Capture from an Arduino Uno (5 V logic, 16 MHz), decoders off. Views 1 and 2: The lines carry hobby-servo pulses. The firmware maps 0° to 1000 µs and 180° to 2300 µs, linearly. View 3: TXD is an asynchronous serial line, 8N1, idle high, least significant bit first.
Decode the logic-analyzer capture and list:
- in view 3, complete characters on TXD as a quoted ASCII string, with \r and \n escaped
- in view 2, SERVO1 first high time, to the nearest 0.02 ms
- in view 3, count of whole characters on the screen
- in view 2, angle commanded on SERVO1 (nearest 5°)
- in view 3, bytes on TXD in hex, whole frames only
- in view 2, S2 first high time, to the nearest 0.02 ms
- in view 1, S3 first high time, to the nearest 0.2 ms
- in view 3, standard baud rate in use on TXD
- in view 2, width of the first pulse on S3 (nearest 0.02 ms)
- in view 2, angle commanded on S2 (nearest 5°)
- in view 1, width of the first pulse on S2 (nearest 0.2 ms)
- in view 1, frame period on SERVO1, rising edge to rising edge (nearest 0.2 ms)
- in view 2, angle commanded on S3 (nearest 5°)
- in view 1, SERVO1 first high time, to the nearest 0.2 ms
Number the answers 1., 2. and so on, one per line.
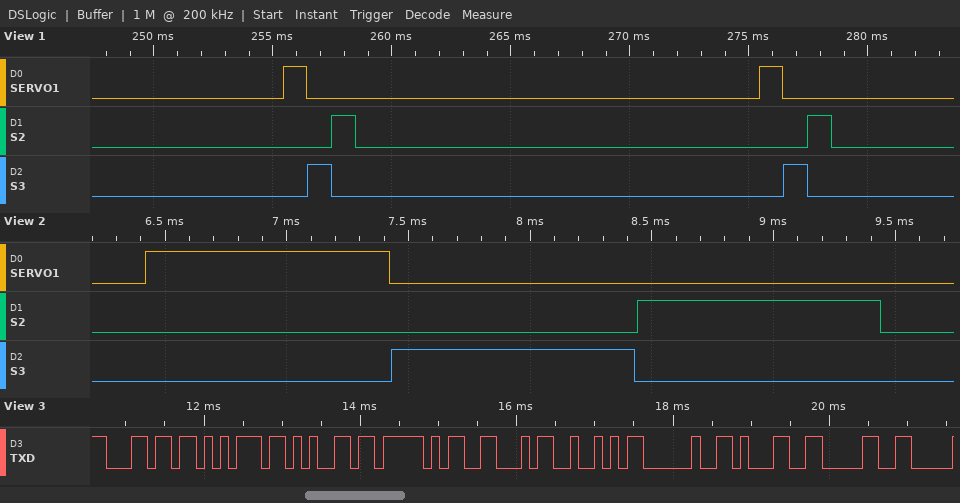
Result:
1. "lue_FR 10"
2. 1.00 ms
3. 9
4. 0°
5. 0x6C 0x75 0x65 0x5F 0x46 0x52 0x20 0x31 0x30
6. 1.00 ms
7. 1.0 ms
8. 9600 baud
9. 1.00 ms
10. 0°
11. 1.0 ms
12. 20.0 ms
13. 0°
14. 1.0 ms
